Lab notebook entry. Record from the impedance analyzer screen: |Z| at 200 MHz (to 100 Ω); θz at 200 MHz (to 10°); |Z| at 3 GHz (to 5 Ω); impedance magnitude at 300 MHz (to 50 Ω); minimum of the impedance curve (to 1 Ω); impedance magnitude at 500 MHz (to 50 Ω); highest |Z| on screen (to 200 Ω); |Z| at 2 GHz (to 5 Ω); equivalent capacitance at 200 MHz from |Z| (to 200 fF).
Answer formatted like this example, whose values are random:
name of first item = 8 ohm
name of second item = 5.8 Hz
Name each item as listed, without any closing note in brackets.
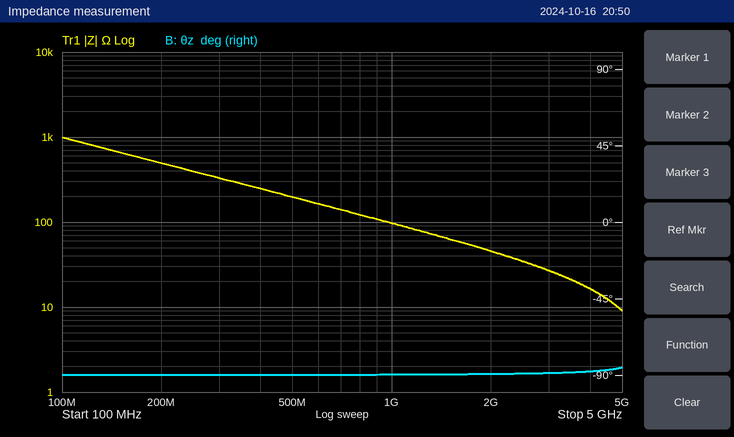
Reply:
|Z| at 200 MHz = 500 Ω
θz at 200 MHz = -90°
|Z| at 3 GHz = 25 Ω
impedance magnitude at 300 MHz = 350 Ω
minimum of the impedance curve = 9 Ω
impedance magnitude at 500 MHz = 200 Ω
highest |Z| on screen = 1.0 kΩ
|Z| at 2 GHz = 45 Ω
equivalent capacitance at 200 MHz from |Z| = 1.6 pF
